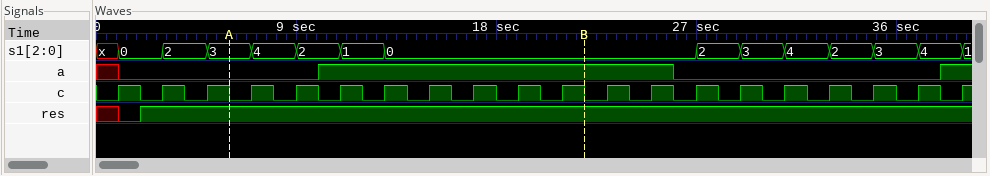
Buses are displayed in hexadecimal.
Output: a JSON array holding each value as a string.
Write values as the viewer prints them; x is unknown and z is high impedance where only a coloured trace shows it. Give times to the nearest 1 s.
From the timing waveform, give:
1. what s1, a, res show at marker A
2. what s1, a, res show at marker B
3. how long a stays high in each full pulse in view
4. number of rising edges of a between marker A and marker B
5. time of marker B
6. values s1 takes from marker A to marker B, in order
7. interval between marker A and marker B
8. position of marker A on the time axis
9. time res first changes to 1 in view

["s1=3, a=0, res=1", "s1=0, a=1, res=1", "16 s", "1", "22 s", "3, 4, 2, 1, 0", "16 s", "6 s", "2 s"]
